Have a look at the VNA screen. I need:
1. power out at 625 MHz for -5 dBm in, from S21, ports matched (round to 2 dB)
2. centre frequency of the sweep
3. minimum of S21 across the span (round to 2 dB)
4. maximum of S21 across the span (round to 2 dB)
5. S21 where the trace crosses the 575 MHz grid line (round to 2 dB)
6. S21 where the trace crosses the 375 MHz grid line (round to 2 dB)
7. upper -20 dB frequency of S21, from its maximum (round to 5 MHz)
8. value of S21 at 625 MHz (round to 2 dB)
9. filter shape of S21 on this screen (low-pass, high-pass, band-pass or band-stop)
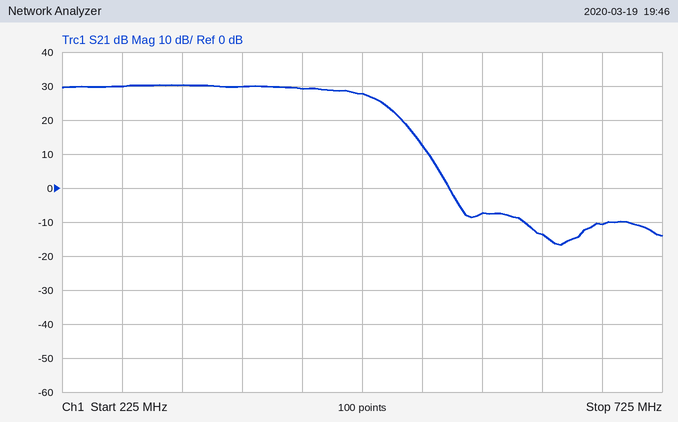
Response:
-18 dBm
475 MHz
-16 dB
30 dB
-8 dB
30 dB
530 MHz
-14 dB
low-pass
